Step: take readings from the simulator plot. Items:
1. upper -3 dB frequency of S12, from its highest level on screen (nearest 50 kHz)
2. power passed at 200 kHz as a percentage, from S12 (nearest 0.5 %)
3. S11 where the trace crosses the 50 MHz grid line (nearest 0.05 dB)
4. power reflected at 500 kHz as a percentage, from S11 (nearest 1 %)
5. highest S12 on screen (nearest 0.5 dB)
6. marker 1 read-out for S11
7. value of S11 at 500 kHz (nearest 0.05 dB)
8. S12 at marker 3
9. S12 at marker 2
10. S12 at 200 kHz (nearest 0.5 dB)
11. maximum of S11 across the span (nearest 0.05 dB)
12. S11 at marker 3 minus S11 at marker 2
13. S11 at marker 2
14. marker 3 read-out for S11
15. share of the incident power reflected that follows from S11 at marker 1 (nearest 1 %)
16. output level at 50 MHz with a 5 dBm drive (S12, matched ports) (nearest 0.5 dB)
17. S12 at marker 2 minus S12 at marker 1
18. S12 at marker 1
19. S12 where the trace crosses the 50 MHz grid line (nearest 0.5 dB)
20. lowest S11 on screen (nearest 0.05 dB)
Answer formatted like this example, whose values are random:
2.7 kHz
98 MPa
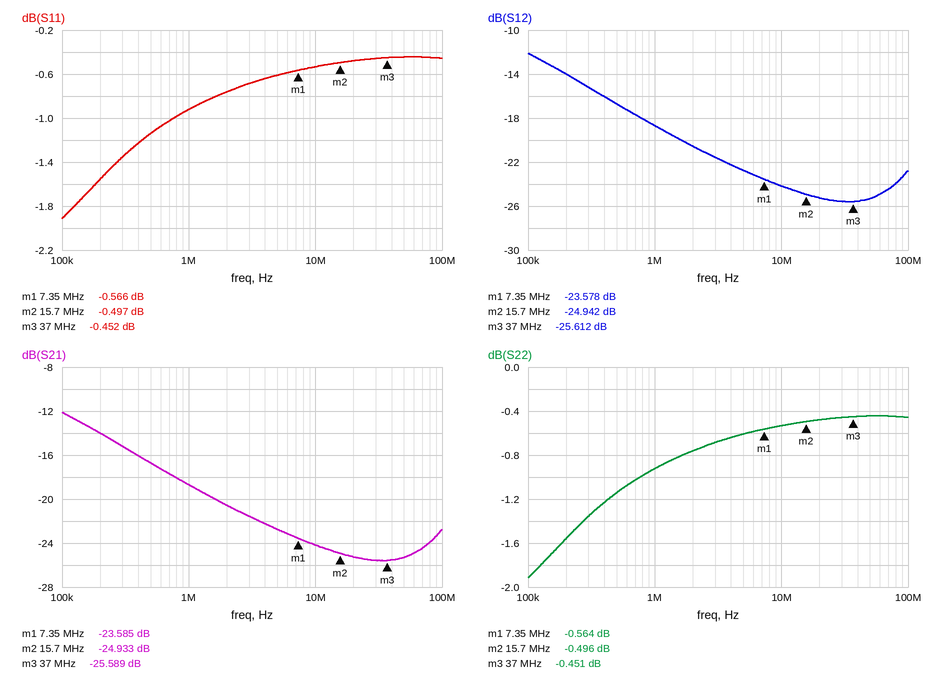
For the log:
300 kHz
4.0 %
-0.45 dB
77 %
-12.0 dB
-0.566 dB
-1.15 dB
-25.612 dB
-24.942 dB
-14.0 dB
-0.45 dB
0.045 dB
-0.497 dB
-0.452 dB
88 %
-20.5 dBm
-1.364 dB
-23.578 dB
-25.5 dB
-1.90 dB
